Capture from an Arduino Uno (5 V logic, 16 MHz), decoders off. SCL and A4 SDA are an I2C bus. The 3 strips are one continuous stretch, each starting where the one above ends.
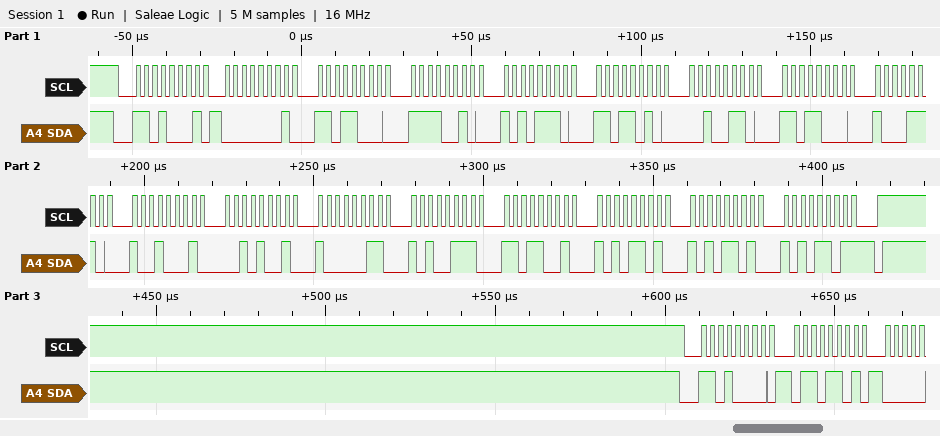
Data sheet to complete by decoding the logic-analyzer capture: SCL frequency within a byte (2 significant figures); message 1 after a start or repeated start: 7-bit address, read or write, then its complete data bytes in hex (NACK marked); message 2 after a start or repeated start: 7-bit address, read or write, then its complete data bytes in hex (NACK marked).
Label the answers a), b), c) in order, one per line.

a) 400 kHz
b) 0x68 read: 01 D8 F2 AE DA 26 D8 8E 91 29 83 A7 D9 AD AD AD NACK
c) 0x68 write: 6D
